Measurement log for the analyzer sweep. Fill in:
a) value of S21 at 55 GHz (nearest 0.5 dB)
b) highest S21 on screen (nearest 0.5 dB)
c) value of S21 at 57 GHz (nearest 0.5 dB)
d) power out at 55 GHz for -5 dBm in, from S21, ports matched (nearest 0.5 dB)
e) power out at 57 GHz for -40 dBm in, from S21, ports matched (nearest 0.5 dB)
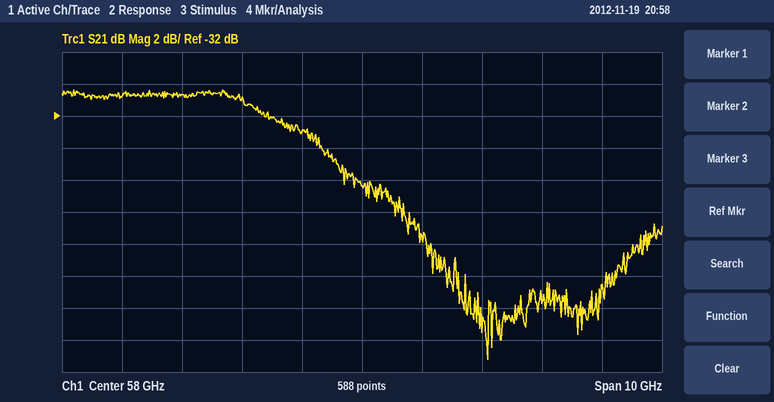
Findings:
-30.5 dB
-30.5 dB
-33.0 dB
-35.5 dBm
-73.0 dBm
